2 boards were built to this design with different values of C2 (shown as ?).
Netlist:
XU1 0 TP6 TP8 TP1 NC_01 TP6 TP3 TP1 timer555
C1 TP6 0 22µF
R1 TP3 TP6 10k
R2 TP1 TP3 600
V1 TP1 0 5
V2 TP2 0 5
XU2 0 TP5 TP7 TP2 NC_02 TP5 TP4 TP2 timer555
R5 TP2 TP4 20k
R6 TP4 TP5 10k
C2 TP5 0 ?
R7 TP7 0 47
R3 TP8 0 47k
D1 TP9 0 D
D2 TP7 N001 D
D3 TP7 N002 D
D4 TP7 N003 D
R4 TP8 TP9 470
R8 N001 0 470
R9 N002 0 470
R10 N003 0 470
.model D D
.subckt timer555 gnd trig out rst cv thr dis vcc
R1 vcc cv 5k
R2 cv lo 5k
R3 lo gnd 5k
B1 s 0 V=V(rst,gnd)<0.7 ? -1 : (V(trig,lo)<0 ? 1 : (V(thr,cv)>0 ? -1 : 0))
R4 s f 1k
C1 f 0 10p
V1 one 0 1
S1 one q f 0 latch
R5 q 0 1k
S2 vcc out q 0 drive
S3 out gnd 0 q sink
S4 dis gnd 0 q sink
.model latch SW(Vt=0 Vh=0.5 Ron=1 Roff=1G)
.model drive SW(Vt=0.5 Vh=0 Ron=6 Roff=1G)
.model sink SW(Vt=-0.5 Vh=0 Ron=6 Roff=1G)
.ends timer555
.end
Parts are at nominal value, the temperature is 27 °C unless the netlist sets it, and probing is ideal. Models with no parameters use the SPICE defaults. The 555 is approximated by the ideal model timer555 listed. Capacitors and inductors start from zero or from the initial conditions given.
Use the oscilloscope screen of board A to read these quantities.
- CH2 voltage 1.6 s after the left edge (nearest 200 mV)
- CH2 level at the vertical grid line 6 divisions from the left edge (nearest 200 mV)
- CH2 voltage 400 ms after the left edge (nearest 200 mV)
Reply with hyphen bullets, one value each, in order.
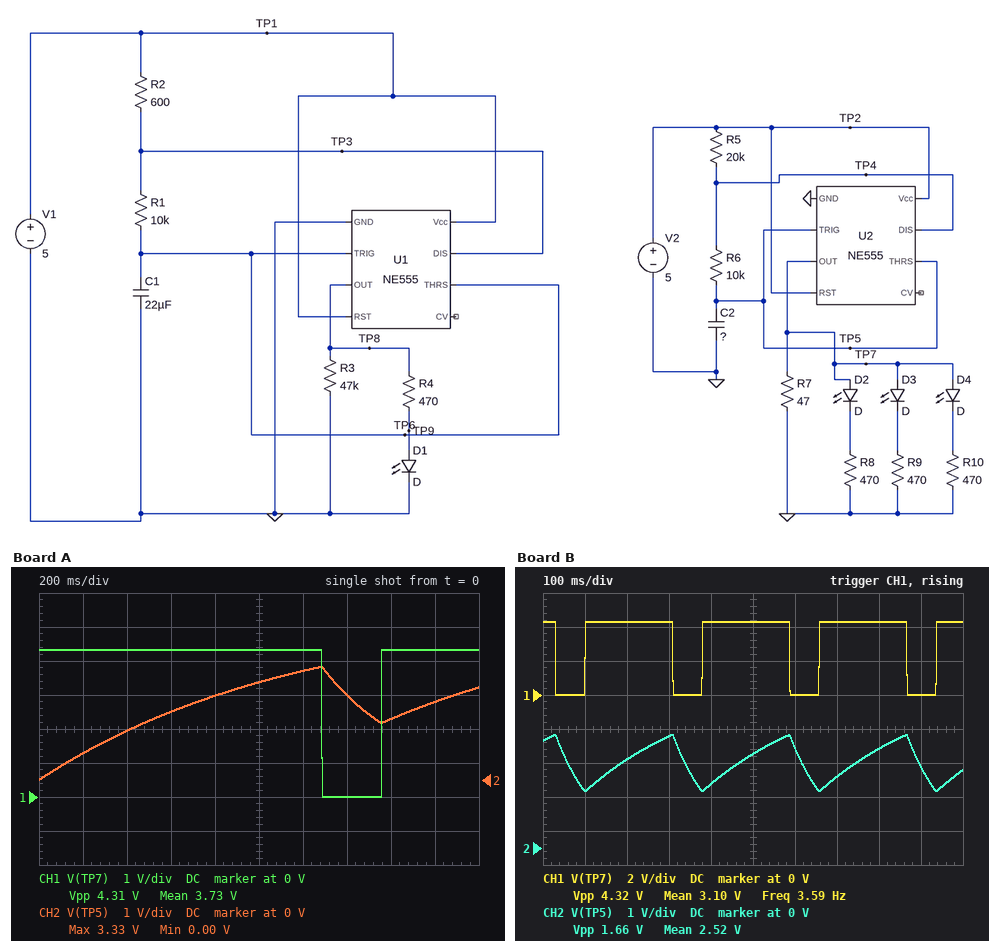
- 1.8 V
- 3.2 V
- 1.4 V
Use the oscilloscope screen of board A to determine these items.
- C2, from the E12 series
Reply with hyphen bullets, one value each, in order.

- 39 µF
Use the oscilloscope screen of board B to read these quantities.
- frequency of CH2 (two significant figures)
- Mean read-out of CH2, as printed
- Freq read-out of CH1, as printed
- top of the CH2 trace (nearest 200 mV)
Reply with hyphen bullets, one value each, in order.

- 3.6 Hz
- 2.52 V
- 3.59 Hz
- 3.4 V
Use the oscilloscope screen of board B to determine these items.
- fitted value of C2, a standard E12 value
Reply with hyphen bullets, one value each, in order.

- 10 µF
